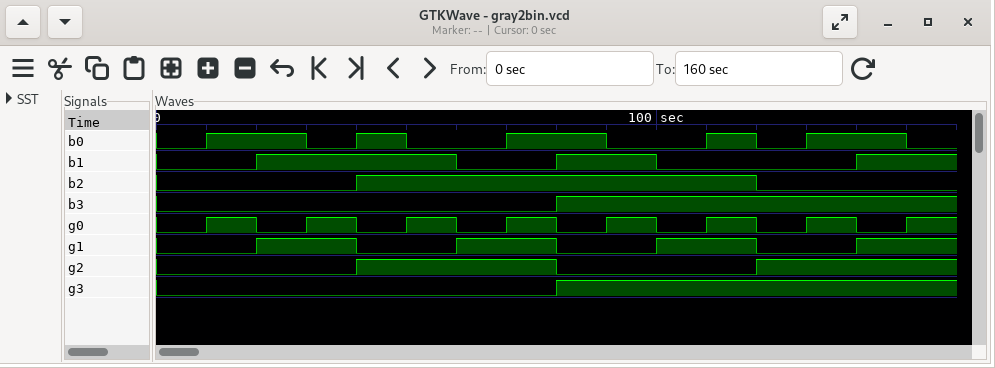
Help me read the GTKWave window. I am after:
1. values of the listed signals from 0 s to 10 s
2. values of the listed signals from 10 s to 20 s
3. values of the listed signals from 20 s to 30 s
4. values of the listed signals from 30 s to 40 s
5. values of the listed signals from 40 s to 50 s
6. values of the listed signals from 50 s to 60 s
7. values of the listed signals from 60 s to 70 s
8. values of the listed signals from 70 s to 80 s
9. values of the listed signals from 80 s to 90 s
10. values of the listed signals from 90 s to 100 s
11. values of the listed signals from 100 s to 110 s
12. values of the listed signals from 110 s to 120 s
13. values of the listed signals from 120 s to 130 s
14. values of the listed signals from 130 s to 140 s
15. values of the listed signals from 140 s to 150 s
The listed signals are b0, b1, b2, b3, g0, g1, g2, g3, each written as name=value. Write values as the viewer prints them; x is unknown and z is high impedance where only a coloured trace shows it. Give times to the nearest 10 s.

b0=0, b1=0, b2=0, b3=0, g0=0, g1=0, g2=0, g3=0
b0=1, b1=0, b2=0, b3=0, g0=1, g1=0, g2=0, g3=0
b0=1, b1=1, b2=0, b3=0, g0=0, g1=1, g2=0, g3=0
b0=0, b1=1, b2=0, b3=0, g0=1, g1=1, g2=0, g3=0
b0=1, b1=1, b2=1, b3=0, g0=0, g1=0, g2=1, g3=0
b0=0, b1=1, b2=1, b3=0, g0=1, g1=0, g2=1, g3=0
b0=0, b1=0, b2=1, b3=0, g0=0, g1=1, g2=1, g3=0
b0=1, b1=0, b2=1, b3=0, g0=1, g1=1, g2=1, g3=0
b0=1, b1=1, b2=1, b3=1, g0=0, g1=0, g2=0, g3=1
b0=0, b1=1, b2=1, b3=1, g0=1, g1=0, g2=0, g3=1
b0=0, b1=0, b2=1, b3=1, g0=0, g1=1, g2=0, g3=1
b0=1, b1=0, b2=1, b3=1, g0=1, g1=1, g2=0, g3=1
b0=0, b1=0, b2=0, b3=1, g0=0, g1=0, g2=1, g3=1
b0=1, b1=0, b2=0, b3=1, g0=1, g1=0, g2=1, g3=1
b0=1, b1=1, b2=0, b3=1, g0=0, g1=1, g2=1, g3=1
